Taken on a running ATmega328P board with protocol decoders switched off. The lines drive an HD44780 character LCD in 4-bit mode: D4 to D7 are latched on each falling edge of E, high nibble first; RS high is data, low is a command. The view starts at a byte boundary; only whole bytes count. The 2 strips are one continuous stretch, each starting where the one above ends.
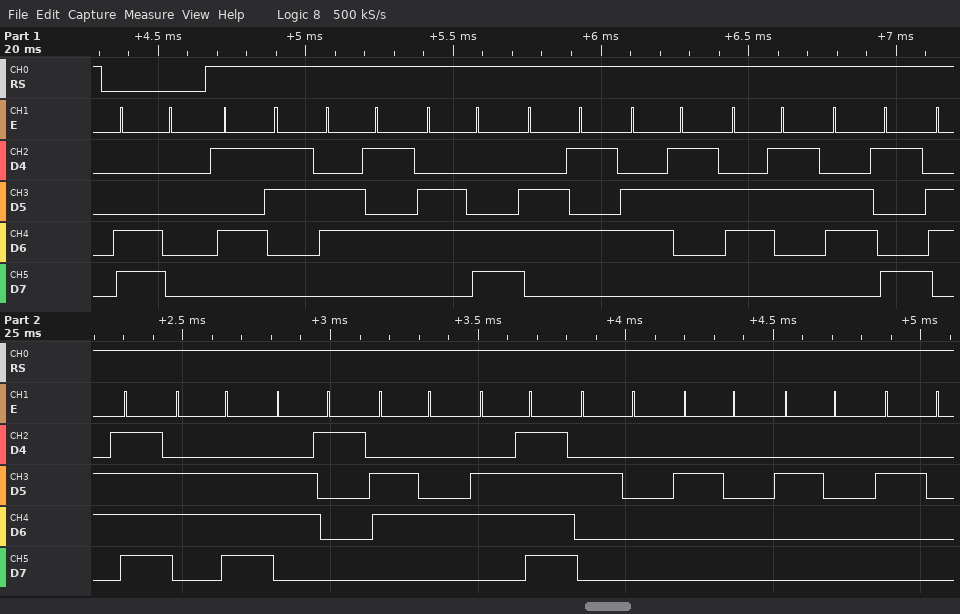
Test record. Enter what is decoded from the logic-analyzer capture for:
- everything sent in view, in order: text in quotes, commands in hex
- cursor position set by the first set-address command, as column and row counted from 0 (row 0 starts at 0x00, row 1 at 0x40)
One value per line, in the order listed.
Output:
0xC0 "Seleccionado    "
column 0, row 1
